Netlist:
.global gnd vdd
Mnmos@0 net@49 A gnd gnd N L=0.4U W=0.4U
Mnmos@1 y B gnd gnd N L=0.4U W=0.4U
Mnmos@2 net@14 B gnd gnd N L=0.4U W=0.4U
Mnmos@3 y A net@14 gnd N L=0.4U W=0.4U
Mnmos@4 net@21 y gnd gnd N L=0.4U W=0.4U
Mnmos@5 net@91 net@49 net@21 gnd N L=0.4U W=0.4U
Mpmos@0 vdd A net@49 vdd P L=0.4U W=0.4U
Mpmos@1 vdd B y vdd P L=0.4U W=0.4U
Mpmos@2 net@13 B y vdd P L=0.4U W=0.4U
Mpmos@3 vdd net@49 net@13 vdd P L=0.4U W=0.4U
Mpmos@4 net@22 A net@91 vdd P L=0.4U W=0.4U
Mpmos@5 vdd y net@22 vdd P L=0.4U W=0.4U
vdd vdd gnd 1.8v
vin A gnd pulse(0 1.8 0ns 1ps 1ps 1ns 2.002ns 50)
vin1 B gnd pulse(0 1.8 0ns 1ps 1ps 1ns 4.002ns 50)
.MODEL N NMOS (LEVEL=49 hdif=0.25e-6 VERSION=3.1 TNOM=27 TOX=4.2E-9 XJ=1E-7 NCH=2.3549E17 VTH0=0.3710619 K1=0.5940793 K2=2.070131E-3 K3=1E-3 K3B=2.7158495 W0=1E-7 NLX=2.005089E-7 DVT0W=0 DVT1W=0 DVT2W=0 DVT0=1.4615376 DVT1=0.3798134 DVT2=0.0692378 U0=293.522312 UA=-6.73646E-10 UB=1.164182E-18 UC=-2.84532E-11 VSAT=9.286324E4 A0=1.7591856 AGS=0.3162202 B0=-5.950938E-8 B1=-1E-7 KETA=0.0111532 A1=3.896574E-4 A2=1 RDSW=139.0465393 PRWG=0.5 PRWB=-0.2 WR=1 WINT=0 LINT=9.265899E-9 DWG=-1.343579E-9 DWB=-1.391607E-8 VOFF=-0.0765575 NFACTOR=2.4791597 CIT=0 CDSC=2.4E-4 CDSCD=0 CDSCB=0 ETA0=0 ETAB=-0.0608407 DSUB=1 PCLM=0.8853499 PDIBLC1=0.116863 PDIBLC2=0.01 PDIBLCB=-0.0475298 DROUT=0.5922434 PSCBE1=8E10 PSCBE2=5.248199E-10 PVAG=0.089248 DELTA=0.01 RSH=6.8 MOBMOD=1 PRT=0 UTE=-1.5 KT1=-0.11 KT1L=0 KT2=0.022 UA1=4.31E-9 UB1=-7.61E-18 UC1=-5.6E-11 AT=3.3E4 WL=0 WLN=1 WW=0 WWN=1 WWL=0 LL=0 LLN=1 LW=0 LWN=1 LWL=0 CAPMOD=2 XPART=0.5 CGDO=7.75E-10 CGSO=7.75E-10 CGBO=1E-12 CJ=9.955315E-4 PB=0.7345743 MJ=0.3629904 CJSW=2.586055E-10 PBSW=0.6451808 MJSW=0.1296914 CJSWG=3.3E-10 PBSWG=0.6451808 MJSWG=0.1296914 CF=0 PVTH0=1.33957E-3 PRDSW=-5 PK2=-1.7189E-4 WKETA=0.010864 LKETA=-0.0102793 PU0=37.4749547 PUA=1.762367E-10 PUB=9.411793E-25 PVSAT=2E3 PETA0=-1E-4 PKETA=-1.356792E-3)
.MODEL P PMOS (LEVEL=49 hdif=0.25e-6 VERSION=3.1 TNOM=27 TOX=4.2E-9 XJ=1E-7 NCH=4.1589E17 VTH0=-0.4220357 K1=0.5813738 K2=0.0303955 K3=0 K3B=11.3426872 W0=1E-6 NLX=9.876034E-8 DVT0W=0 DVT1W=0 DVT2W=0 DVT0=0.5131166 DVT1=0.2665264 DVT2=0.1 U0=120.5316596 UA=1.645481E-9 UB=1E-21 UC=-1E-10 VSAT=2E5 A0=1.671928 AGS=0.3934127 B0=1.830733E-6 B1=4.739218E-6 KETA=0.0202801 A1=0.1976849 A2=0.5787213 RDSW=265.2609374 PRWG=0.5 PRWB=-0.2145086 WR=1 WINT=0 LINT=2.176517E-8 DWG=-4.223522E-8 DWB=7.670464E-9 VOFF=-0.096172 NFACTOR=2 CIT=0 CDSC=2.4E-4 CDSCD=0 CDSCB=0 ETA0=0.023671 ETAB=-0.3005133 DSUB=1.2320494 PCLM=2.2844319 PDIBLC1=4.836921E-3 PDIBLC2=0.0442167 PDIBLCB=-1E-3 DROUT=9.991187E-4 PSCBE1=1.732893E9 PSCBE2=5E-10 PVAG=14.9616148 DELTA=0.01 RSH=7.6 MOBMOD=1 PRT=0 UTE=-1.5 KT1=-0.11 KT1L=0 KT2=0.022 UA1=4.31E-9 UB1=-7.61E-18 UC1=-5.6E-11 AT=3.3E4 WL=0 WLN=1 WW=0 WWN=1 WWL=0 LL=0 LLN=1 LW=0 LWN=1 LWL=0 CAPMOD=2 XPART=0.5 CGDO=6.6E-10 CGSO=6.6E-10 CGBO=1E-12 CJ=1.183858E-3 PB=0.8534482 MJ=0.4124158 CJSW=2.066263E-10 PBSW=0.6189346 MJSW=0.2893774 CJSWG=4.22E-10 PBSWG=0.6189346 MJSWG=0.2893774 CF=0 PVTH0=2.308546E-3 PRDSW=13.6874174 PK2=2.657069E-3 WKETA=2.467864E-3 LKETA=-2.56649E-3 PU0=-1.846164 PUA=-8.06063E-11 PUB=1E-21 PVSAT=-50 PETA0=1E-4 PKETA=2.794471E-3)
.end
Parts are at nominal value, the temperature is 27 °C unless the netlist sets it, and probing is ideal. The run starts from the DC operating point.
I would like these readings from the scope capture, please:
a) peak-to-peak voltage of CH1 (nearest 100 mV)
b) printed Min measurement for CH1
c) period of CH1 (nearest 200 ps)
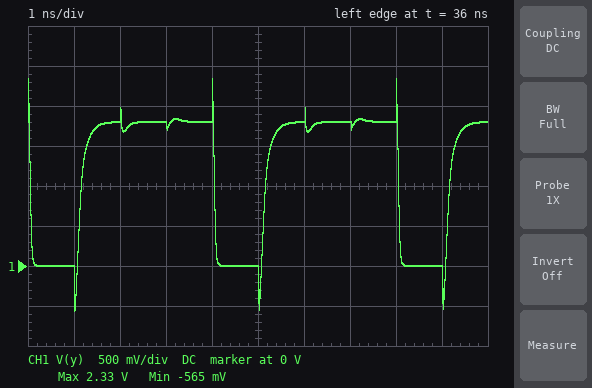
2.9 V
-565 mV
4.0 ns
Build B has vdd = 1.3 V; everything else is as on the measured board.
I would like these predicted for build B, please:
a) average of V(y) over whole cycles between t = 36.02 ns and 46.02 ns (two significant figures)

860 mV
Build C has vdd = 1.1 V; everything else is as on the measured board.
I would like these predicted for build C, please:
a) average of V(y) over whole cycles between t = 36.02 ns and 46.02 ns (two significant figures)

670 mV
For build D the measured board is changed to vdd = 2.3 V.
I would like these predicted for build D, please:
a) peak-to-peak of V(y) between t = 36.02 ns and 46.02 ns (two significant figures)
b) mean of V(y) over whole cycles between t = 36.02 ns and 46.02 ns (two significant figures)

3.4 V
1.7 V
